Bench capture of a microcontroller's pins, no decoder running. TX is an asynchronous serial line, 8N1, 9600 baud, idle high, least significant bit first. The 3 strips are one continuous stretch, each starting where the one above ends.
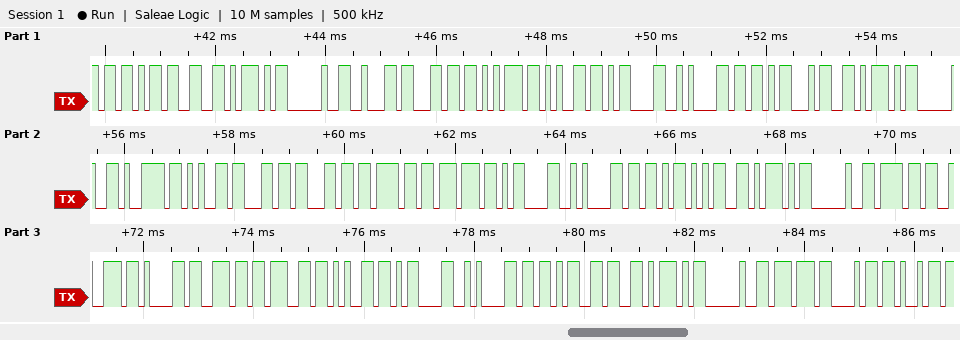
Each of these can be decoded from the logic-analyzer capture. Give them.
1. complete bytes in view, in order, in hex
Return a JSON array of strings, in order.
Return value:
["0x5B 0x33 0x5D 0x20 0x62 0x6C 0x75 0x65 0x0D 0x0A 0x5B 0x34 0x5D 0x20 0x79 0x65 0x6C 0x6C 0x6F 0x77 0x0D 0x0A 0x5B 0x35 0x5D 0x20 0x6F 0x72 0x61 0x6E 0x67 0x65 0x0D 0x0A 0x5B 0x36 0x5D 0x20 0x77 0x68 0x69"]
